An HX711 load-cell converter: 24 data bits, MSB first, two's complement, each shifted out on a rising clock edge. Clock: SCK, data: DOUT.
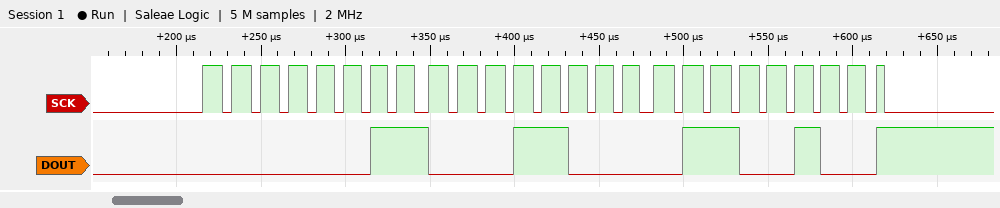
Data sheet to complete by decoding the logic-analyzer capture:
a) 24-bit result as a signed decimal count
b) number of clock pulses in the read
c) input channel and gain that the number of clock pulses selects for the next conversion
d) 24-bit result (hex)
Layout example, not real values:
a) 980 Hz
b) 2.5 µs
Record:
a) 202852
b) 25
c) channel A, gain 128
d) 0x031864
